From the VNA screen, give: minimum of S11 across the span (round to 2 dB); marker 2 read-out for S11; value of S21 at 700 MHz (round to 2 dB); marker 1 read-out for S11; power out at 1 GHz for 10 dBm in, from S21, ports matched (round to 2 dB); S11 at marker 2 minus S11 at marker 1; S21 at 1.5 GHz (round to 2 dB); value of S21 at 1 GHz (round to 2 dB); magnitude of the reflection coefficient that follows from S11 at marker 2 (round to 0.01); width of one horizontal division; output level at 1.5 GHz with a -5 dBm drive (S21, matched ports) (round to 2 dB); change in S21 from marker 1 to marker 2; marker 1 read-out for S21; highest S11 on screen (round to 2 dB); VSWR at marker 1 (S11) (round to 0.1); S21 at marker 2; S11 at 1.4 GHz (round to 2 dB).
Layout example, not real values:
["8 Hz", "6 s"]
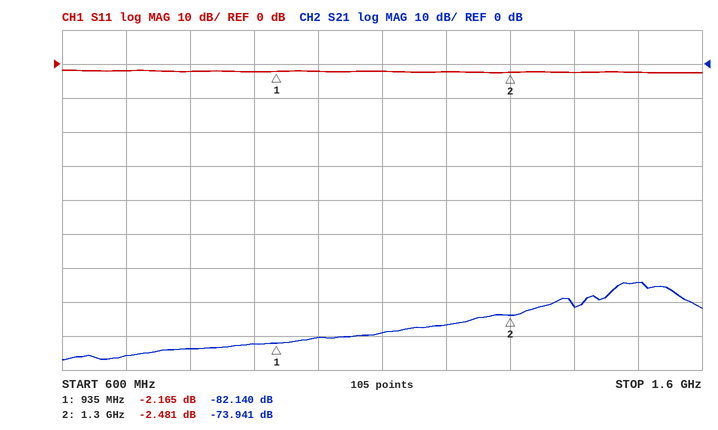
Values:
["-2 dB", "-2.481 dB", "-86 dB", "-2.165 dB", "-70 dBm", "-0.316 dB", "-64 dB", "-80 dB", "0.75", "100 MHz", "-70 dBm", "8.199 dB", "-82.140 dB", "-2 dB", "8.1", "-73.941 dB", "-2 dB"]
